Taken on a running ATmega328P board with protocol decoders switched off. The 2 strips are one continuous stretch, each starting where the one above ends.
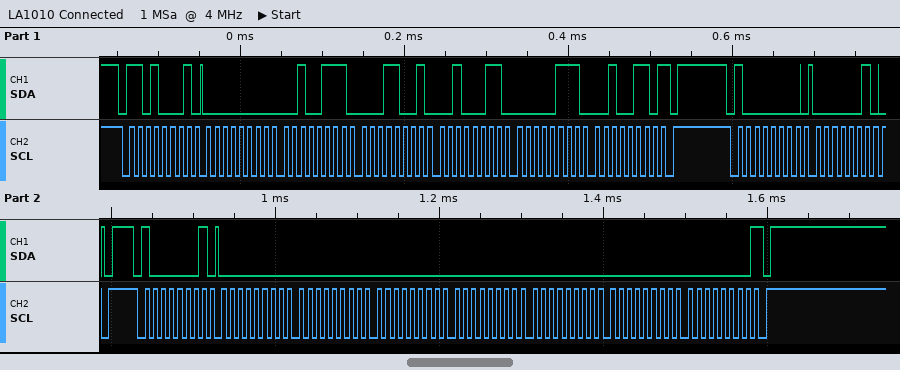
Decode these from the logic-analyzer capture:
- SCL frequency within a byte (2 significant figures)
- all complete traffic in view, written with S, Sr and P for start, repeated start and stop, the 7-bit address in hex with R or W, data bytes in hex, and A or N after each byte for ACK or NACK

100 kHz
S 68R A 00 A 27 A 19 A 23 A 07 A 26 N P S 40W A 02 A P S 40R A 00 A 00 A 00 A 00 A 00 A 00 A 00 N P
